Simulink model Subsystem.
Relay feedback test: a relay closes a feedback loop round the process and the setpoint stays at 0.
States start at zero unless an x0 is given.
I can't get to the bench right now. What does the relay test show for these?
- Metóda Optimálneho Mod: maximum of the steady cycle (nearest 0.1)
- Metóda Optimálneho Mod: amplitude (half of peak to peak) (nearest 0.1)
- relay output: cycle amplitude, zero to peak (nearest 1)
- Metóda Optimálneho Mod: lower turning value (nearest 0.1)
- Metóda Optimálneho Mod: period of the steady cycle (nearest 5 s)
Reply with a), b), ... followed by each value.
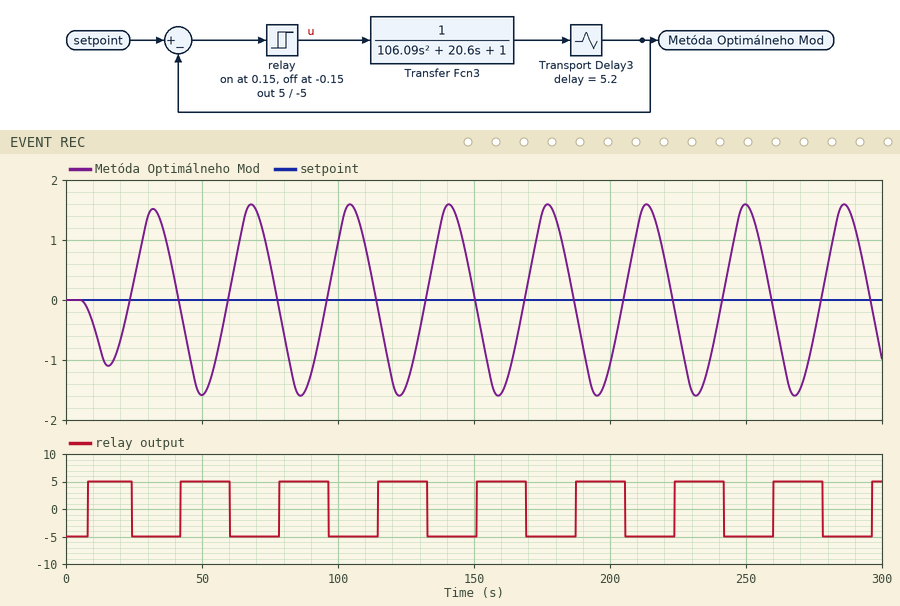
a) 1.6
b) 1.6
c) 5
d) -1.6
e) 35 s
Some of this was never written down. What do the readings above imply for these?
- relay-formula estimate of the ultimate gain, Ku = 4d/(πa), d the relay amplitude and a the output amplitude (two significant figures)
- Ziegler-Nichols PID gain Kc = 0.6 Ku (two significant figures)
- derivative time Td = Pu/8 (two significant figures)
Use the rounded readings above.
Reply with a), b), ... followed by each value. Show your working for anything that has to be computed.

a) 4 × 5 / (π × 1.6) = 4.0
b) 0.6 × 4 = 2.4
c) 35 / 8 = 4.4 s
